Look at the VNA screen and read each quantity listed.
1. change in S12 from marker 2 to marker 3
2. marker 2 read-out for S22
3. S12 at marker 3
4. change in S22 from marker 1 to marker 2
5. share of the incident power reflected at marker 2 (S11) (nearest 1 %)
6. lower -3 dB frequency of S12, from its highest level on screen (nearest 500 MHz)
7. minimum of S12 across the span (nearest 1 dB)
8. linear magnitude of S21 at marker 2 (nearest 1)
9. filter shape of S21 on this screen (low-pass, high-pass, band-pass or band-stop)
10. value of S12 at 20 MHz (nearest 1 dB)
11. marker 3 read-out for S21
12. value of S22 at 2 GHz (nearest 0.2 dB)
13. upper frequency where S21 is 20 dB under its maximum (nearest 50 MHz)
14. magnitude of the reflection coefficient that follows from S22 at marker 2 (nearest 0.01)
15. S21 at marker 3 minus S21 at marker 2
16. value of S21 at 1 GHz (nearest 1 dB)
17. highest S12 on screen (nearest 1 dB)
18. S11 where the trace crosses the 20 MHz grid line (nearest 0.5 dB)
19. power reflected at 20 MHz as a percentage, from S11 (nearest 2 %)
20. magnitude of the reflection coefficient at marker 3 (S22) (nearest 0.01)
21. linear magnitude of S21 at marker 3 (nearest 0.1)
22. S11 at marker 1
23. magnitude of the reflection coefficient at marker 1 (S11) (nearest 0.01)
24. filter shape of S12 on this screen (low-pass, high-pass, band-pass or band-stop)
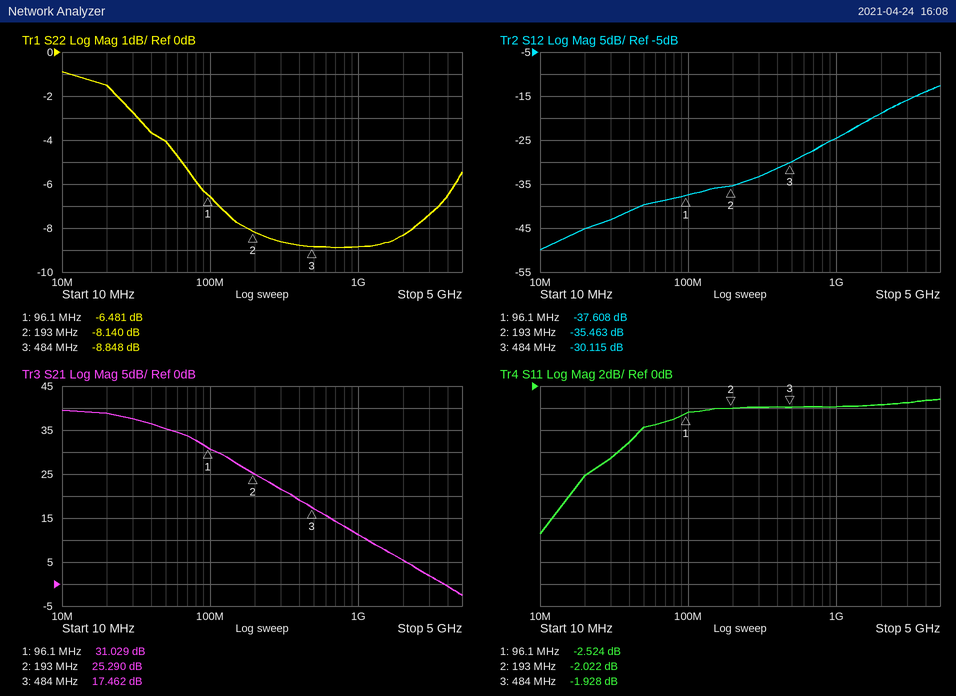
5.348 dB
-8.140 dB
-30.115 dB
-1.659 dB
63 %
3.0 GHz
-50 dB
18
low-pass
-45 dB
17.462 dB
-8.4 dB
400 MHz
0.39
-7.828 dB
11 dB
-13 dB
-8.0 dB
16 %
0.36
7.5
-2.524 dB
0.75
high-pass
